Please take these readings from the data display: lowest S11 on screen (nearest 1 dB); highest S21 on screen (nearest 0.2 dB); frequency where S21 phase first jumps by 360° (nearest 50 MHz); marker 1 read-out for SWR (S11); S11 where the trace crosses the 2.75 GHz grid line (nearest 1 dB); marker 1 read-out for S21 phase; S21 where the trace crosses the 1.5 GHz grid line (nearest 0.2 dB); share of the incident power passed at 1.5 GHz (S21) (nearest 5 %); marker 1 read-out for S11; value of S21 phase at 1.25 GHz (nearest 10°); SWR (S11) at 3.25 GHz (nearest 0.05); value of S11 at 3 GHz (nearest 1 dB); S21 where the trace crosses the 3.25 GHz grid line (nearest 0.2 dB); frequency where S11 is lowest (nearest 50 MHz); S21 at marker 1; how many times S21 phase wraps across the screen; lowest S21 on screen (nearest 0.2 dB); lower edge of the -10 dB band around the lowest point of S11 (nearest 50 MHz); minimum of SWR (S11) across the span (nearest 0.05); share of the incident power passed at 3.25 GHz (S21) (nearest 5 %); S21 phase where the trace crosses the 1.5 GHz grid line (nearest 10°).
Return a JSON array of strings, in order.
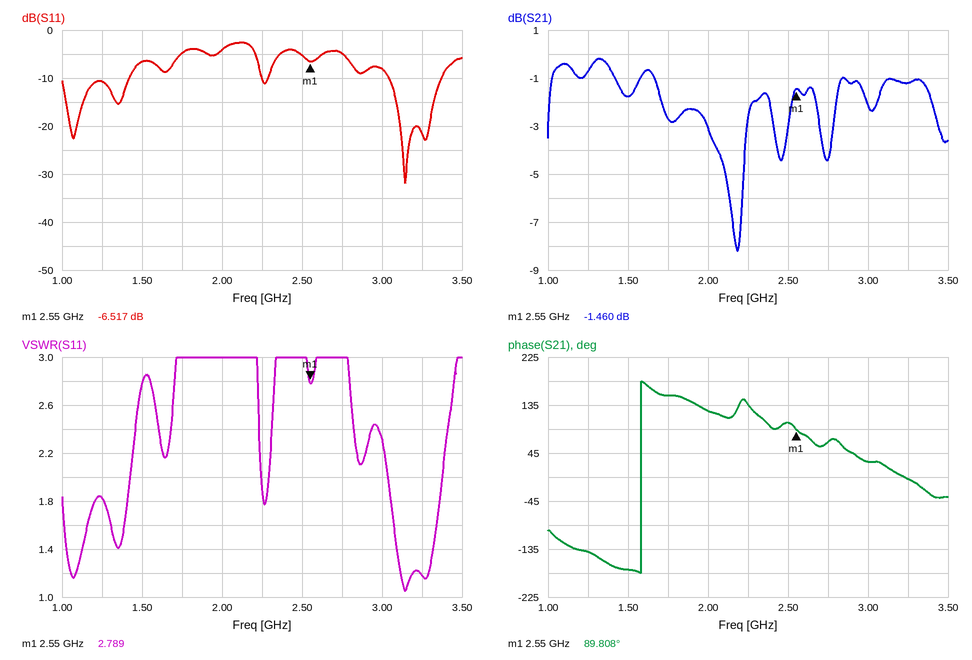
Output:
["-32 dB", "-0.2 dB", "1.60 GHz", "2.789", "-5 dB", "89.808°", "-1.8 dB", "65 %", "-6.517 dB", "-140°", "1.20", "-8 dB", "-1.2 dB", "3.15 GHz", "-1.460 dB", "1", "-8.2 dB", "3.05 GHz", "1.05", "75 %", "-170°"]
